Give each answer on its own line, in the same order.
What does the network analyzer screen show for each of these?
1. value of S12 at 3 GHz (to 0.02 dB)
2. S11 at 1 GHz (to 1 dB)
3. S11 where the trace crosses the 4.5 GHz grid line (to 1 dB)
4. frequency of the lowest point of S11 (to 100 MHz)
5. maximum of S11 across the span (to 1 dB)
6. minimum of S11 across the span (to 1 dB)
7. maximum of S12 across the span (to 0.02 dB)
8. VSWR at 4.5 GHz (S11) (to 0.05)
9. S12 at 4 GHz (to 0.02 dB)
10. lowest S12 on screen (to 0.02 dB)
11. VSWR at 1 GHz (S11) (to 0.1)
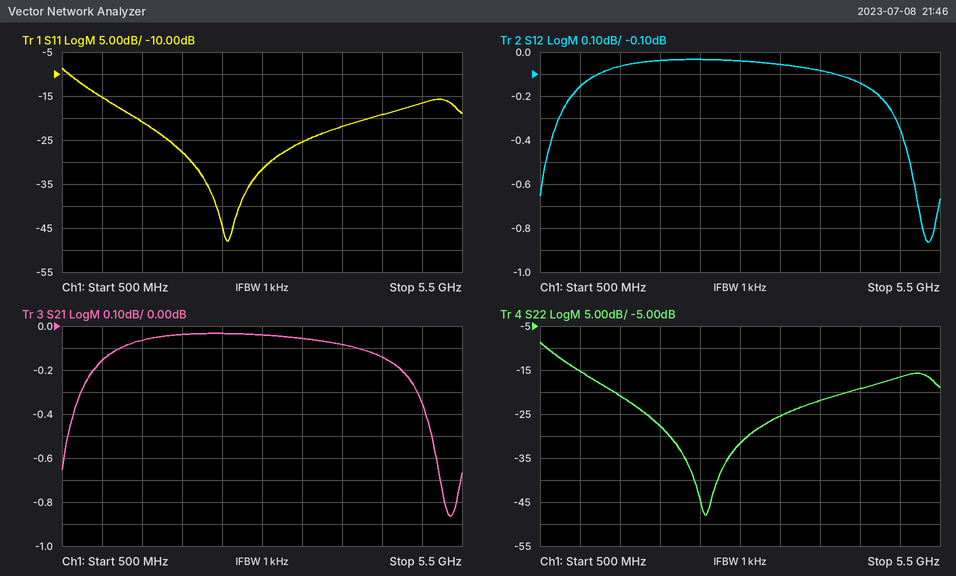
-0.04 dB
-15 dB
-19 dB
2.6 GHz
-9 dB
-48 dB
-0.04 dB
1.25
-0.08 dB
-0.86 dB
1.4
